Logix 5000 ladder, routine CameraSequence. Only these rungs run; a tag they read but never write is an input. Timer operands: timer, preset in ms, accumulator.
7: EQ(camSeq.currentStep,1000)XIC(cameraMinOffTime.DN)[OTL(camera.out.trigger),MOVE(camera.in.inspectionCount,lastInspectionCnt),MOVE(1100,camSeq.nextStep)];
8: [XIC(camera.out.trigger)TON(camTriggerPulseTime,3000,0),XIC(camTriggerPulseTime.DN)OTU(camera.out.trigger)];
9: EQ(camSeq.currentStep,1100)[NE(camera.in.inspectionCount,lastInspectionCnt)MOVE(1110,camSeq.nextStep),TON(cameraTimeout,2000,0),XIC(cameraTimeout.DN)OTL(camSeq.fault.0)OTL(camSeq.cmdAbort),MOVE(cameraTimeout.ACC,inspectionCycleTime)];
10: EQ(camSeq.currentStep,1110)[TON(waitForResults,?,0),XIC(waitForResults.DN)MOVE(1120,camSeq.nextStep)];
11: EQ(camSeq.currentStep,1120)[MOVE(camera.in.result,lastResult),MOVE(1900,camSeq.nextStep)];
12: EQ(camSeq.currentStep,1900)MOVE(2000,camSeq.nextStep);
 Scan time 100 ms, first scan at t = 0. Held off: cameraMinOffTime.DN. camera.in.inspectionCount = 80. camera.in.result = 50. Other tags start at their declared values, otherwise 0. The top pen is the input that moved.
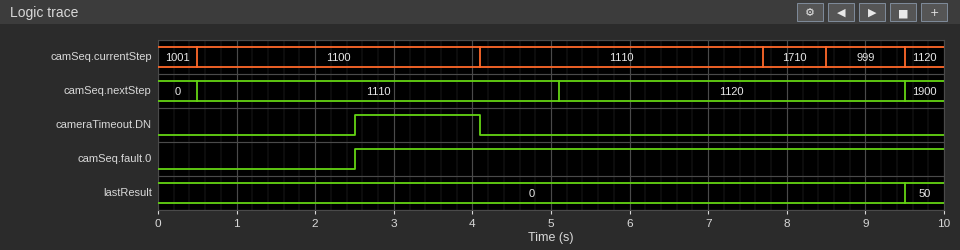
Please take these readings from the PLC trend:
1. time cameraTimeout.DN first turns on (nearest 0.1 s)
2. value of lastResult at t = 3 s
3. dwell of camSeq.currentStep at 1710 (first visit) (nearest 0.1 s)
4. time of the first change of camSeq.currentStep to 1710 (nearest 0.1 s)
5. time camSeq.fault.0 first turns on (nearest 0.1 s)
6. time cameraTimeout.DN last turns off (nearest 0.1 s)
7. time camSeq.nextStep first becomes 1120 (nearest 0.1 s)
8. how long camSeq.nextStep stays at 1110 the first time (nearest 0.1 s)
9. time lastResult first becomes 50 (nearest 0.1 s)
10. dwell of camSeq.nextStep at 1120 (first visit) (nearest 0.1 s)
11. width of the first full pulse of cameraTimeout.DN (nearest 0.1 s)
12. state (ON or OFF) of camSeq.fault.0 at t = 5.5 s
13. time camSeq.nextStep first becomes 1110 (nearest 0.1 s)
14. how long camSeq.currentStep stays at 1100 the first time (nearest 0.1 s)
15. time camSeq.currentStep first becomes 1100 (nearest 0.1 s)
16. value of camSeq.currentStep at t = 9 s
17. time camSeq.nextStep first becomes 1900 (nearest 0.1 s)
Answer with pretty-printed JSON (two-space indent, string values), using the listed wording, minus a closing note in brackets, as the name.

{
  "time cameraTimeout.DN first turns on": "2.5 s",
  "value of lastResult at t = 3 s": "0",
  "dwell of camSeq.currentStep at 1710 (first visit)": "0.8 s",
  "time of the first change of camSeq.currentStep to 1710": "7.7 s",
  "time camSeq.fault.0 first turns on": "2.5 s",
  "time cameraTimeout.DN last turns off": "4.1 s",
  "time camSeq.nextStep first becomes 1120": "5.1 s",
  "how long camSeq.nextStep stays at 1110 the first time": "4.6 s",
  "time lastResult first becomes 50": "9.5 s",
  "dwell of camSeq.nextStep at 1120 (first visit)": "4.4 s",
  "width of the first full pulse of cameraTimeout.DN": "1.6 s",
  "state (ON or OFF) of camSeq.fault.0 at t = 5.5 s": "ON",
  "time camSeq.nextStep first becomes 1110": "0.5 s",
  "how long camSeq.currentStep stays at 1100 the first time": "3.6 s",
  "time camSeq.currentStep first becomes 1100": "0.5 s",
  "value of camSeq.currentStep at t = 9 s": "999",
  "time camSeq.nextStep first becomes 1900": "9.5 s"
}
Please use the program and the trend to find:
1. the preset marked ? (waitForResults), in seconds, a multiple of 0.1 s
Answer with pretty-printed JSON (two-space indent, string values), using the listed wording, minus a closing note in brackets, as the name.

{
  "the preset marked ? (waitForResults), in seconds, a multiple of 0.1 s": "1.0 s"
}
